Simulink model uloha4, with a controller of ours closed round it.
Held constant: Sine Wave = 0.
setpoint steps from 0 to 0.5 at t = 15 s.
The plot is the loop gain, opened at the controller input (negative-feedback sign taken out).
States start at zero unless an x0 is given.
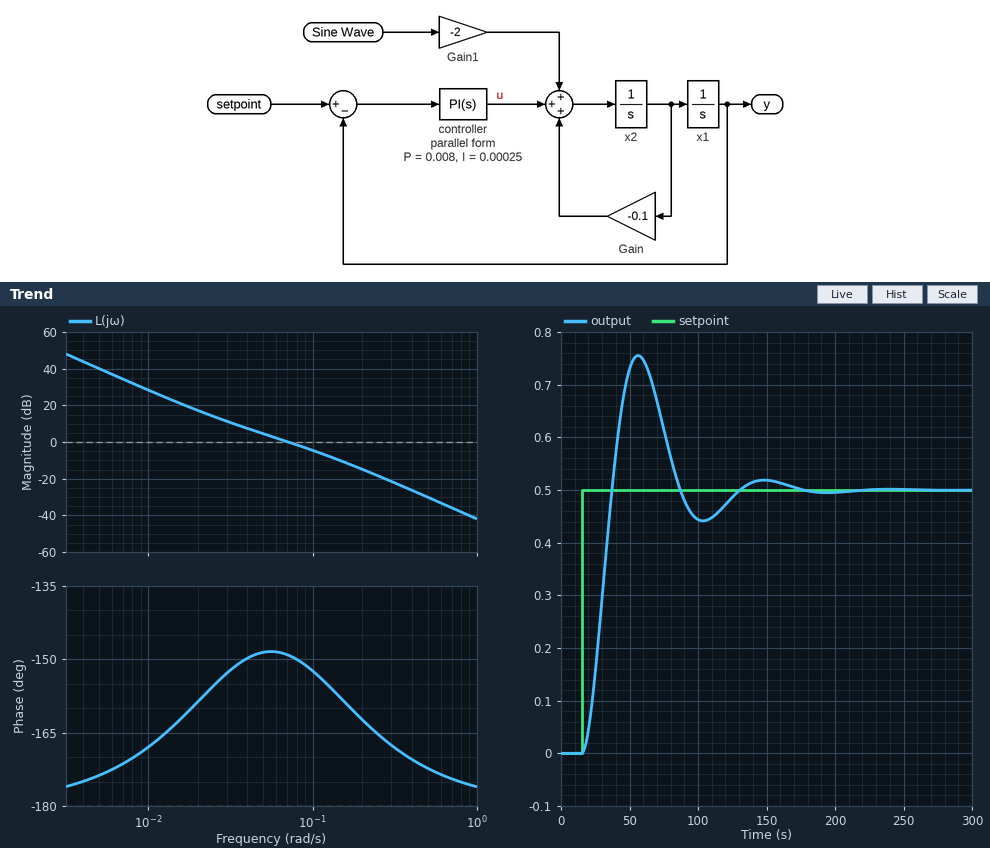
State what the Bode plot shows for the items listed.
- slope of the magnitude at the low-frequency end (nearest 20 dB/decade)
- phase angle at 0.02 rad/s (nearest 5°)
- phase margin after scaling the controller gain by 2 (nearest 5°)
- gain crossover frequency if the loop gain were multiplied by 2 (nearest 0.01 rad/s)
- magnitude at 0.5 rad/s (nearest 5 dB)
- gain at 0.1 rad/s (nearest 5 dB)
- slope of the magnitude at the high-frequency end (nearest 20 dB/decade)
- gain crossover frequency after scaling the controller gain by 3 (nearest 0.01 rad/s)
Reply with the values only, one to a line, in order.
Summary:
-40 dB/decade
-160°
25°
0.11 rad/s
-30 dB
-5 dB
-40 dB/decade
0.14 rad/s
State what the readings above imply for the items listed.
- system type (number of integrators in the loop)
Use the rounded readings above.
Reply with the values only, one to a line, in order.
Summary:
2
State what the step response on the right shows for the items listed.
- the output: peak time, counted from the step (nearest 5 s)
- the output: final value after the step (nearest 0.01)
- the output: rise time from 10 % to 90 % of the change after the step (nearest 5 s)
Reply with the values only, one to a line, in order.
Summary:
40 s
0.50
15 s
